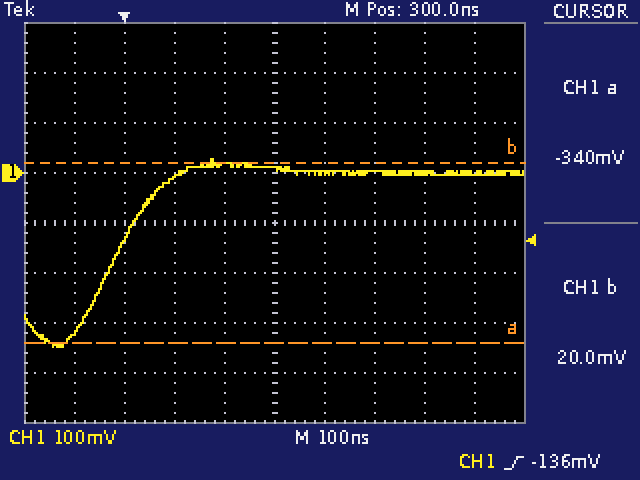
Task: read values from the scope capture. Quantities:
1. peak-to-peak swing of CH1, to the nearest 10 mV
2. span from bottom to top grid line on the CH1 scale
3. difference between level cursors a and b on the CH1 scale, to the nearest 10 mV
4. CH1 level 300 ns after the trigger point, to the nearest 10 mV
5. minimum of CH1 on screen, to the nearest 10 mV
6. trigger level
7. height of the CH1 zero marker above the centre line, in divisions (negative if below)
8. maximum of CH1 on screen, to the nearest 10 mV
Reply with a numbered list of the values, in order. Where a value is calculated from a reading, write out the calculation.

1. 30 mV − (-350 mV) = 380 mV
2. 800 mV
3. 360 mV
4. 10 mV
5. -350 mV
6. -136 mV
7. +1.0 div
8. 30 mV
